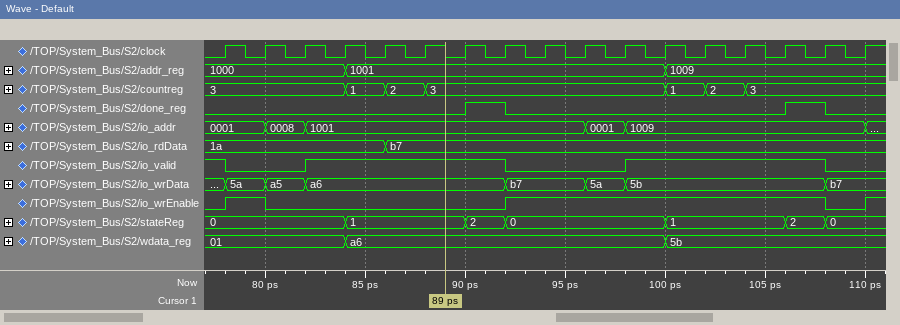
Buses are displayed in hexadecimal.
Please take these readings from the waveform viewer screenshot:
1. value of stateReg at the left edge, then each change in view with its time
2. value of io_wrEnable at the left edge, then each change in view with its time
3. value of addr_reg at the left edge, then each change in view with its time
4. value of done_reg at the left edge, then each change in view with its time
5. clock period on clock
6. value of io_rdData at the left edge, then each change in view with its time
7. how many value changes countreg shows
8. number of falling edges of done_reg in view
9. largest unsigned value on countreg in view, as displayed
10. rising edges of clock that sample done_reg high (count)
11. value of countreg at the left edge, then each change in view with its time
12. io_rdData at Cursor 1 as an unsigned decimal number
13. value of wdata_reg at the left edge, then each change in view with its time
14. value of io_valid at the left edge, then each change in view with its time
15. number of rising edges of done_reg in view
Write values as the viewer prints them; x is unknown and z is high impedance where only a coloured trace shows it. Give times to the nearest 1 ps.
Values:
0, 1 at 84 ps, 2 at 90 ps, 0 at 92 ps, 1 at 100 ps, 2 at 106 ps, 0 at 108 ps
0, 1 at 78 ps, 0 at 80 ps, 1 at 92 ps, 0 at 108 ps, 1 at 110 ps
1000, 1001 at 84 ps, 1009 at 100 ps
0, 1 at 90 ps, 0 at 92 ps, 1 at 106 ps, 0 at 108 ps
2 ps
1a, b7 at 86 ps
6
2
3
2
3, 1 at 84 ps, 2 at 86 ps, 3 at 88 ps, 1 at 100 ps, 2 at 102 ps, 3 at 104 ps
183
01, a6 at 84 ps, 5b at 100 ps
1, 0 at 78 ps, 1 at 82 ps, 0 at 92 ps, 1 at 98 ps, 0 at 108 ps
2
